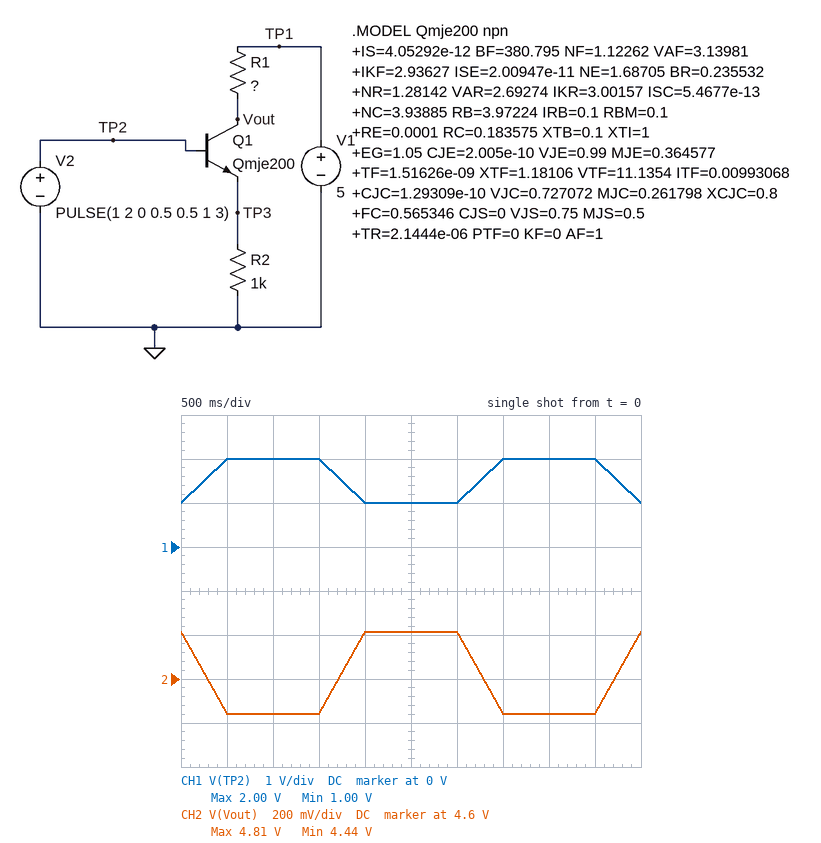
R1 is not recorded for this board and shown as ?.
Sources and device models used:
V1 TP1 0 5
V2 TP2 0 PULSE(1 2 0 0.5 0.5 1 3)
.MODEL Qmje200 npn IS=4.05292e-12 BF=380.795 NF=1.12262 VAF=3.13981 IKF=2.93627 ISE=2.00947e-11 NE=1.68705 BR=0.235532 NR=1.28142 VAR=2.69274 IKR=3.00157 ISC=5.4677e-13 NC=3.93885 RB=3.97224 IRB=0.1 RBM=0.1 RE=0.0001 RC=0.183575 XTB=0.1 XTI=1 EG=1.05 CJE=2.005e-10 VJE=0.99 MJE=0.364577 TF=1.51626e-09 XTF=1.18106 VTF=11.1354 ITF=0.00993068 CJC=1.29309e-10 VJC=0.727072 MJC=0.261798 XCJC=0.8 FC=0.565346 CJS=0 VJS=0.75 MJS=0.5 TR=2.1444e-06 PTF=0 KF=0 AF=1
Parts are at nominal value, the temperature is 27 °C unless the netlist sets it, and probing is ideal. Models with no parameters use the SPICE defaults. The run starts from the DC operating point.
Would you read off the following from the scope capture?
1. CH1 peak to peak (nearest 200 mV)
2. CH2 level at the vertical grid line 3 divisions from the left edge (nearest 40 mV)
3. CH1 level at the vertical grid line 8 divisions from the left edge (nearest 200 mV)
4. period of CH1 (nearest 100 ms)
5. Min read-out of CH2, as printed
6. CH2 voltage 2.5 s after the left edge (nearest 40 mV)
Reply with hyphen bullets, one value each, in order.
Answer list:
- 1.0 V
- 4.44 V
- 2.0 V
- 3.0 s
- 4.44 V
- 4.80 V
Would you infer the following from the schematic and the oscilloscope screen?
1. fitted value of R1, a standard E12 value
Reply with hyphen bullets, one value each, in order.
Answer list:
- 390 Ω
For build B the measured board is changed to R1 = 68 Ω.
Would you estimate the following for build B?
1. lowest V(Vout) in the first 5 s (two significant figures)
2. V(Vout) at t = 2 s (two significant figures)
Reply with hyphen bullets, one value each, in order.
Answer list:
- 4.9 V
- 5.0 V
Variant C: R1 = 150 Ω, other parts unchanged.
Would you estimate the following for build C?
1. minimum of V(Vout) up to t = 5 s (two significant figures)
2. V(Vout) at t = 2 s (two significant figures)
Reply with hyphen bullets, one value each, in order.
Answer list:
- 4.8 V
- 4.9 V
